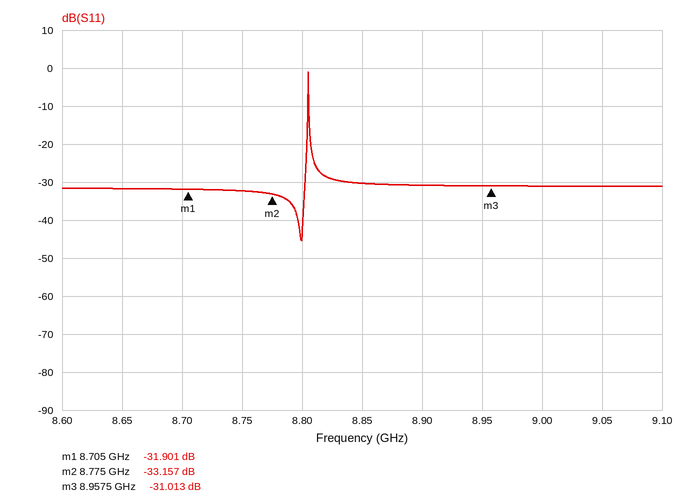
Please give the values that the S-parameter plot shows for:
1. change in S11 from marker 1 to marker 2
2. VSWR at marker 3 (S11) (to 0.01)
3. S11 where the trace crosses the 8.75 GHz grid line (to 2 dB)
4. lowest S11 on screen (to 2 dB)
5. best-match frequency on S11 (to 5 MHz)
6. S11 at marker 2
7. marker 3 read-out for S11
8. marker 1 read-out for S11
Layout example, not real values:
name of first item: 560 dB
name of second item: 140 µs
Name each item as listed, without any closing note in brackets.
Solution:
change in S11 from marker 1 to marker 2: -1.256 dB
VSWR at marker 3 (S11): 1.06
S11 where the trace crosses the 8.75 GHz grid line: -32 dB
lowest S11 on screen: -46 dB
best-match frequency on S11: 8.800 GHz
S11 at marker 2: -33.157 dB
marker 3 read-out for S11: -31.013 dB
marker 1 read-out for S11: -31.901 dB
